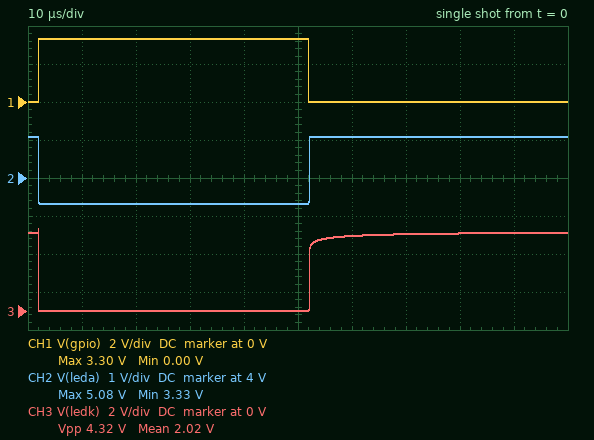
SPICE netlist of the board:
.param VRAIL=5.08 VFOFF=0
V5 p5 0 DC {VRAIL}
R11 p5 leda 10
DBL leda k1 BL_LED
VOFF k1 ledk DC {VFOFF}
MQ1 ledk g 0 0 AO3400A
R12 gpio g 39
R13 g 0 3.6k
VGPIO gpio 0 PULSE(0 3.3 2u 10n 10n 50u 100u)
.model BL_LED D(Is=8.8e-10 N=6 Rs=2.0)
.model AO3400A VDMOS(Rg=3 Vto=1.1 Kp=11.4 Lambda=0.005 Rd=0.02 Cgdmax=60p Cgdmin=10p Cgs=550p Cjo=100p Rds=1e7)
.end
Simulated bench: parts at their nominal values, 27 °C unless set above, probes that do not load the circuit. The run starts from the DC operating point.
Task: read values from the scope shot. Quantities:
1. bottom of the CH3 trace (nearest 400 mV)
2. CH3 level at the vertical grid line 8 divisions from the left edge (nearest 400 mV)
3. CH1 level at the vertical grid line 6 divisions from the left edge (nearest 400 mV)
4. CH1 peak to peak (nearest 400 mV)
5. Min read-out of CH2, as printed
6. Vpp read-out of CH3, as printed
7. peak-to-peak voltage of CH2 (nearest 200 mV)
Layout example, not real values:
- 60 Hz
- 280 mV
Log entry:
- 0 V
- 4.0 V
- 0 V
- 3.2 V
- 3.33 V
- 4.32 V
- 1.8 V
